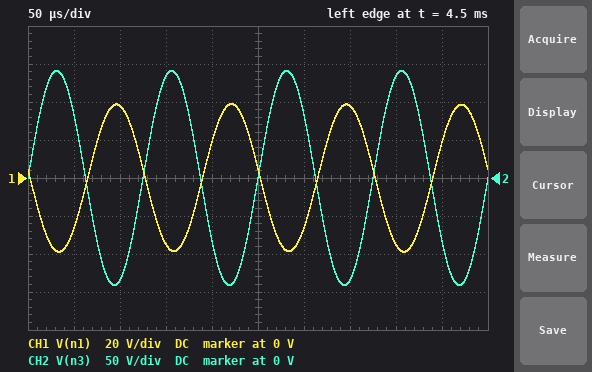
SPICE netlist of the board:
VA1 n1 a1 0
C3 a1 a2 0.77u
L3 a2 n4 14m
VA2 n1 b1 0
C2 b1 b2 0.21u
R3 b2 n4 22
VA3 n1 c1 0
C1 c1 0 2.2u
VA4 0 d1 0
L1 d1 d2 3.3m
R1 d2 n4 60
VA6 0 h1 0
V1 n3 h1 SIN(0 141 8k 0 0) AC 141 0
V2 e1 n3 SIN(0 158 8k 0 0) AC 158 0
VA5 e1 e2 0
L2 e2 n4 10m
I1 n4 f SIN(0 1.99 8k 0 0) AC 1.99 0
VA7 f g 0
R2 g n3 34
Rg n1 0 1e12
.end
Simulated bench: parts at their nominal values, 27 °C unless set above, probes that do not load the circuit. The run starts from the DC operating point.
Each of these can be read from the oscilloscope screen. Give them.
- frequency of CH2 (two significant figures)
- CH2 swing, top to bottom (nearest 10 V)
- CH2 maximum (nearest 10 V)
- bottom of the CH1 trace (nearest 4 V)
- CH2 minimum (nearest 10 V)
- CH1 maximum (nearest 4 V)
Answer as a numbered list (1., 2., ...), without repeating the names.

1. 8.0 kHz
2. 280 V
3. 140 V
4. -40 V
5. -140 V
6. 40 V
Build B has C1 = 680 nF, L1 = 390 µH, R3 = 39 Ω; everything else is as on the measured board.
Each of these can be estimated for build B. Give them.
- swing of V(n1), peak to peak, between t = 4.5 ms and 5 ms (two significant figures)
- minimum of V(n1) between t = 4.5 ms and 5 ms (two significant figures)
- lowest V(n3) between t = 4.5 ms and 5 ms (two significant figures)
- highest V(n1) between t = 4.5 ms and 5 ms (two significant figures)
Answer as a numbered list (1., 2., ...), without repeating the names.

1. 48 V
2. -24 V
3. -140 V
4. 24 V
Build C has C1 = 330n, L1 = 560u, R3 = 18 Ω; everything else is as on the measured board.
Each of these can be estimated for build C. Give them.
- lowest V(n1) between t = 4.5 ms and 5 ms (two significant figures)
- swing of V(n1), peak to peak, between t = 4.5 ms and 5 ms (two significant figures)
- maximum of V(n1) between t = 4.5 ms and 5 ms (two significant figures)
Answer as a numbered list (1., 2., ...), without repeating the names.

1. -50 V
2. 100 V
3. 50 V
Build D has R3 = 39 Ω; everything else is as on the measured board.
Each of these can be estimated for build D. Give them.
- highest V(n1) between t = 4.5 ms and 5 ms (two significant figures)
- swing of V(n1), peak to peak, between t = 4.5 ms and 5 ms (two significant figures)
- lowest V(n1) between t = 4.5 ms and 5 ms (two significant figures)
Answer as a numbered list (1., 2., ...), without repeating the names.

1. 29 V
2. 57 V
3. -29 V
